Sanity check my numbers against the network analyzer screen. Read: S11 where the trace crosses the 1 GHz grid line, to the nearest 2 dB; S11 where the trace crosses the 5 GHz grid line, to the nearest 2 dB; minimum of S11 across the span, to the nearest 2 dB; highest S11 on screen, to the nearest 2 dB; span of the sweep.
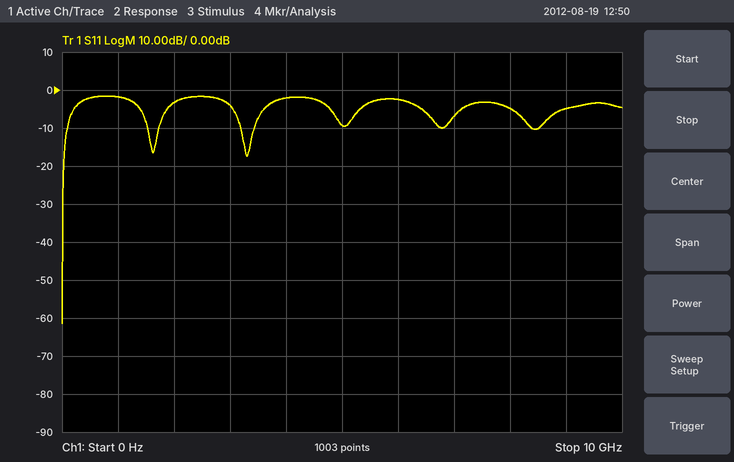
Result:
-2 dB
-10 dB
-62 dB
-2 dB
10 GHz
